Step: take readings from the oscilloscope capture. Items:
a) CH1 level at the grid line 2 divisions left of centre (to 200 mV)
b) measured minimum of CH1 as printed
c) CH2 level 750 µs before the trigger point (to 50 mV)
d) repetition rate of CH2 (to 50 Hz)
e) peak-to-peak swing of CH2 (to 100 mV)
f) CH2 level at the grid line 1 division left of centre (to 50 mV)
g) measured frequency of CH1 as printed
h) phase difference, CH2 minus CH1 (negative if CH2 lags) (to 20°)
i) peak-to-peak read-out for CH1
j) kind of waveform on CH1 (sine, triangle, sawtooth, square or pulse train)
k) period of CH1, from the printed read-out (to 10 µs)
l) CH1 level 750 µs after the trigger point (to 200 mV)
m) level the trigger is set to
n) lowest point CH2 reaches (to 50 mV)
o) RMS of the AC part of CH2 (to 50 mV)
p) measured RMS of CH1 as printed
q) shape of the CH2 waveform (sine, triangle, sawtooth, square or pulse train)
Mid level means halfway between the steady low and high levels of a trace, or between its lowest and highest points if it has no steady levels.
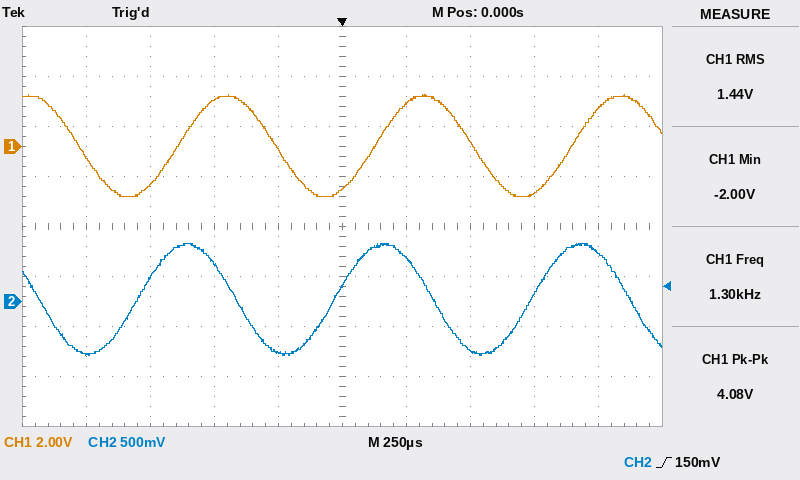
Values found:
1.8 V
-2.00 V
250 mV
1.30 kHz
1.10 V
-500 mV
1.30 kHz
+80°
4.08 V
sine
770 µs
-1.8 V
150 mV
-550 mV
400 mV
1.44 V
sine
